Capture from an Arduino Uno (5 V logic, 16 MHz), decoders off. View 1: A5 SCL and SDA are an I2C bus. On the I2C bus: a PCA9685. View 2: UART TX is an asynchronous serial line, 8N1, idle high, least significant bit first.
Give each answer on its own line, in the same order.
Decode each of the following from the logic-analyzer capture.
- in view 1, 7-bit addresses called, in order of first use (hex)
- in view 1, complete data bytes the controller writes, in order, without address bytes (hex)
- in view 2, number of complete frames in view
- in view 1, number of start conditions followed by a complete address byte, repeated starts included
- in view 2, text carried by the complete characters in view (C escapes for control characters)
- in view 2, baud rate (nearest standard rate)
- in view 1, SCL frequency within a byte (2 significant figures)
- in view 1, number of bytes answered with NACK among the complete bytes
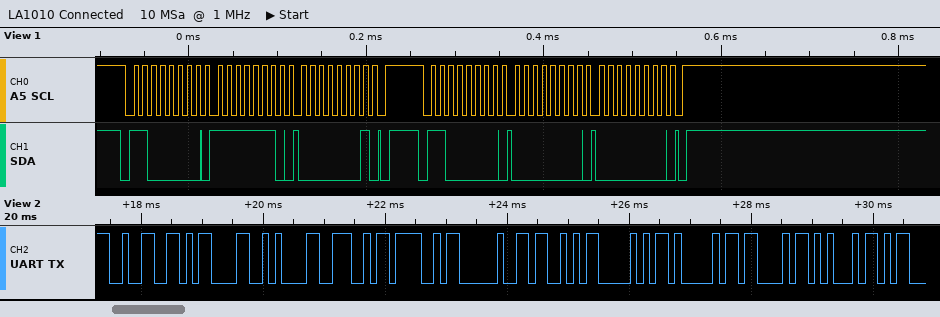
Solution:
0x60
FE 01 00 00
11
2
"2\r\nNO SPACE"
9600 baud
100 kHz
0
